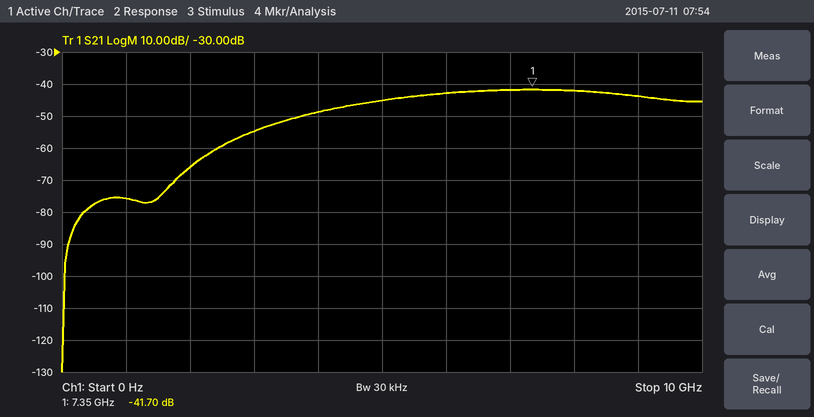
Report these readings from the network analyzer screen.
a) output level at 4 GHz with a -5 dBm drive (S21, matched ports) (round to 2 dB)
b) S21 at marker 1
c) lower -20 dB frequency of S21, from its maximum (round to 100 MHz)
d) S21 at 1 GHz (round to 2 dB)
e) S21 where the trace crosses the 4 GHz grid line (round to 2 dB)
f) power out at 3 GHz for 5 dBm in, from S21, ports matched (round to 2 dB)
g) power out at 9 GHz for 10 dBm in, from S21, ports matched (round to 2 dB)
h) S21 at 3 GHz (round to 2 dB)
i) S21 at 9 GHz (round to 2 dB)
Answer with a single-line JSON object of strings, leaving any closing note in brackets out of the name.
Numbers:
{"output level at 4 GHz with a -5 dBm drive (S21, matched ports)": "-54 dBm", "S21 at marker 1": "-41.70 dB", "lower -20 dB frequency of S21, from its maximum": "2.3 GHz", "S21 at 1 GHz": "-76 dB", "S21 where the trace crosses the 4 GHz grid line": "-48 dB", "power out at 3 GHz for 5 dBm in, from S21, ports matched": "-50 dBm", "power out at 9 GHz for 10 dBm in, from S21, ports matched": "-34 dBm", "S21 at 3 GHz": "-54 dB", "S21 at 9 GHz": "-44 dB"}
